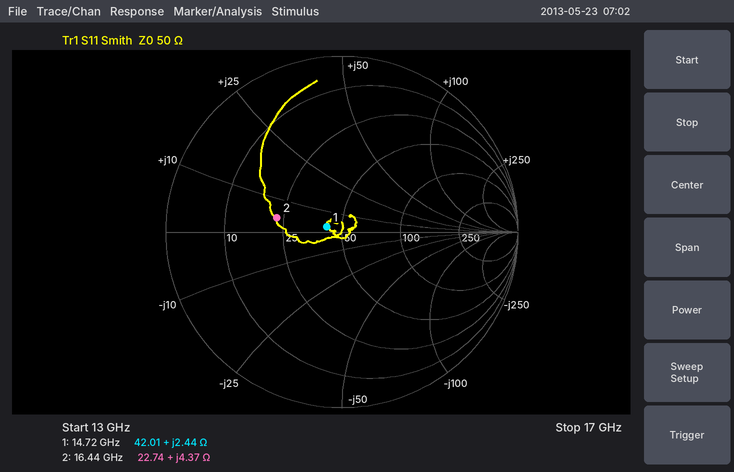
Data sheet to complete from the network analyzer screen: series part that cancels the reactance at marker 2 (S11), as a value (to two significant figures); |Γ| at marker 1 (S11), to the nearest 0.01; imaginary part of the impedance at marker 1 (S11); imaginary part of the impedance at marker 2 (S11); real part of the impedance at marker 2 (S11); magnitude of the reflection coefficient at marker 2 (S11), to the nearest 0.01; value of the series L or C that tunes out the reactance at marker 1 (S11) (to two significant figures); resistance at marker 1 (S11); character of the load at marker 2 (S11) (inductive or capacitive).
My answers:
2.2 pF
0.09
+2.44 Ω
+4.37 Ω
22.74 Ω
0.38
4.4 pF
42.01 Ω
inductive
